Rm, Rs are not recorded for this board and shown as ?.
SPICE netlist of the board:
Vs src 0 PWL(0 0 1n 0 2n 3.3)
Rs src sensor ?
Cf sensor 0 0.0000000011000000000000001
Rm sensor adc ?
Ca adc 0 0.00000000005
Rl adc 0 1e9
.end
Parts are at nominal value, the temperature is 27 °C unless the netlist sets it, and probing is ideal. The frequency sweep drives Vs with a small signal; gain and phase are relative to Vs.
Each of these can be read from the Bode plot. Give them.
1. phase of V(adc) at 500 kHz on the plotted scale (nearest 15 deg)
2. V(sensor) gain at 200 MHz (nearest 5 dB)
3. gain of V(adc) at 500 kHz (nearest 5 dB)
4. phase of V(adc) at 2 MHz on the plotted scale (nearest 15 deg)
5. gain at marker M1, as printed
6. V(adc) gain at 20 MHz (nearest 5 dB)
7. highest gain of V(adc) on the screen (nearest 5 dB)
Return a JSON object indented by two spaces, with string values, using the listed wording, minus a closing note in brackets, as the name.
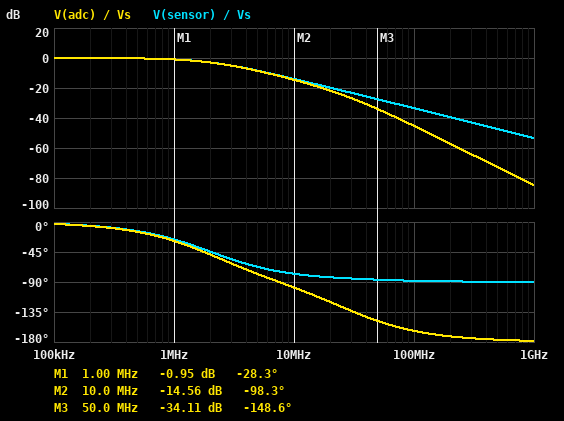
{
  "phase of V(adc) at 500 kHz on the plotted scale": "-15 deg",
  "V(sensor) gain at 200 MHz": "-40 dB",
  "gain of V(adc) at 500 kHz": "0 dB",
  "phase of V(adc) at 2 MHz on the plotted scale": "-45 deg",
  "gain at marker M1, as printed": "-0.95 dB",
  "V(adc) gain at 20 MHz": "-20 dB",
  "highest gain of V(adc) on the screen": "0 dB"
}
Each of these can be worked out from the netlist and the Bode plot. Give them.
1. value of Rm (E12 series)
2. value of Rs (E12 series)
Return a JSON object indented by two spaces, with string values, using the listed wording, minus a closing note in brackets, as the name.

{
  "value of Rm": "120 Ω",
  "value of Rs": "68 Ω"
}
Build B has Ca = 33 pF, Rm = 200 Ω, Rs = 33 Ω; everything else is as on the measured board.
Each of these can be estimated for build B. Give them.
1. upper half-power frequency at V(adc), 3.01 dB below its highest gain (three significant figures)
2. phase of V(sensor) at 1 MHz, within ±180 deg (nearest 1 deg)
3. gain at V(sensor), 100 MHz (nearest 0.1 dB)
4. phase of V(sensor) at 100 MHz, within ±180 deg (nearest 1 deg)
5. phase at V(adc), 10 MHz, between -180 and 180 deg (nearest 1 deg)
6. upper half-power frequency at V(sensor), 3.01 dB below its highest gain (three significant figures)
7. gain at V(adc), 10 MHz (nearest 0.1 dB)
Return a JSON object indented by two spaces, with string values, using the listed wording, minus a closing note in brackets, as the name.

{
  "upper half-power frequency at V(adc), 3.01 dB below its highest gain": "4.12 MHz",
  "phase of V(sensor) at 1 MHz, within ±180 deg": "-13 deg",
  "gain at V(sensor), 100 MHz": "-27.2 dB",
  "phase of V(sensor) at 100 MHz, within ±180 deg": "-87 deg",
  "phase at V(adc), 10 MHz, between -180 and 180 deg": "-89 deg",
  "upper half-power frequency at V(sensor), 3.01 dB below its highest gain": "4.24 MHz",
  "gain at V(adc), 10 MHz": "-8.8 dB"
}
